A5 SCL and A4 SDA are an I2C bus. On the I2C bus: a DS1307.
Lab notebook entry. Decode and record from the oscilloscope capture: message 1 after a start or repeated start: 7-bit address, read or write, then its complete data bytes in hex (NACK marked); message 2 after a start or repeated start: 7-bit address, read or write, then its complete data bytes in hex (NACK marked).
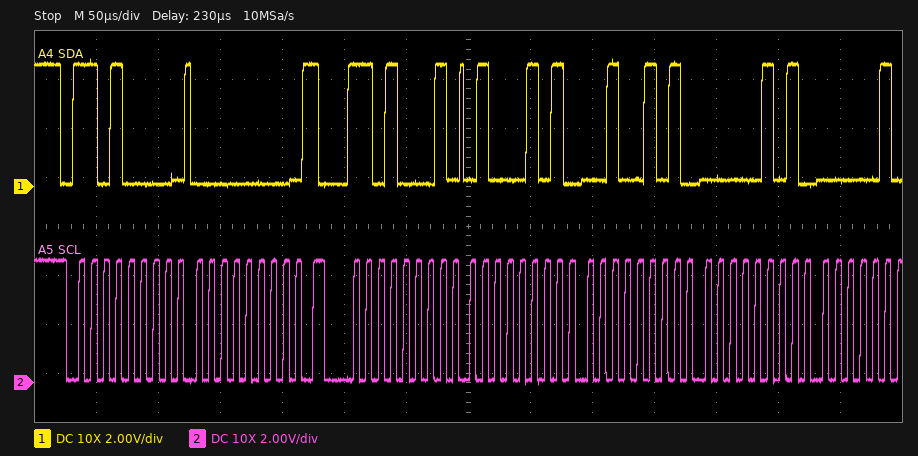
0x68 write: 00
0x68 read: 45 25 05
